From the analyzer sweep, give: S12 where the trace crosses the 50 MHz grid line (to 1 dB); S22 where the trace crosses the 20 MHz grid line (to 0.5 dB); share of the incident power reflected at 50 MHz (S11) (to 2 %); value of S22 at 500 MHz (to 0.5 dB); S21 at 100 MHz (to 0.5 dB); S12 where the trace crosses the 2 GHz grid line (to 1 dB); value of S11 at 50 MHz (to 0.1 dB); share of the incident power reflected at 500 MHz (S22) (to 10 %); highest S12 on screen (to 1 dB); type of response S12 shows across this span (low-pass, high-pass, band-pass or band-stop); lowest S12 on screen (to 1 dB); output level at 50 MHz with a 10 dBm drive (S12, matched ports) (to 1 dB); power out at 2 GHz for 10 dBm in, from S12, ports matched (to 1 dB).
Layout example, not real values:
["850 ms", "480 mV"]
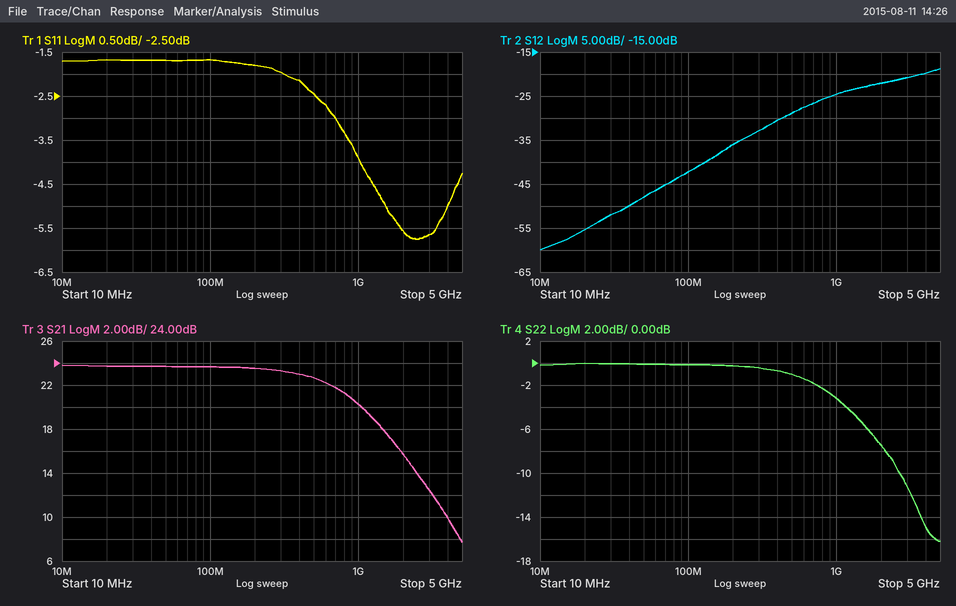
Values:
["-48 dB", "0.0 dB", "68 %", "-1.0 dB", "23.5 dB", "-22 dB", "-1.7 dB", "80 %", "-19 dB", "high-pass", "-60 dB", "-38 dBm", "-12 dBm"]
